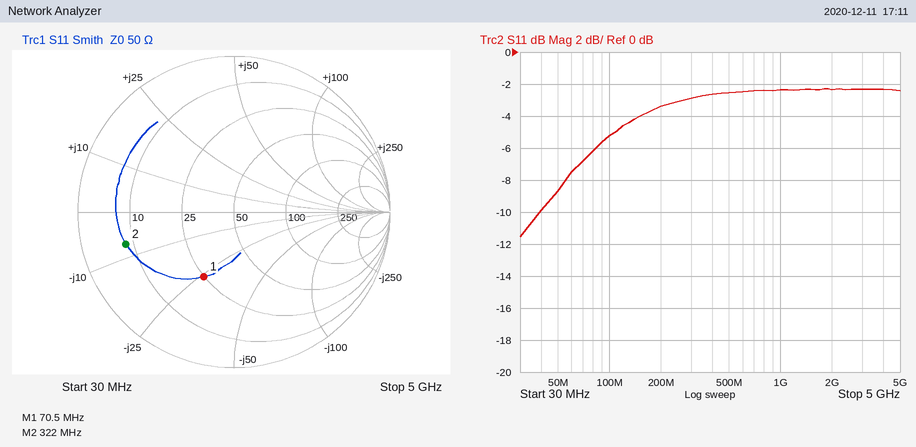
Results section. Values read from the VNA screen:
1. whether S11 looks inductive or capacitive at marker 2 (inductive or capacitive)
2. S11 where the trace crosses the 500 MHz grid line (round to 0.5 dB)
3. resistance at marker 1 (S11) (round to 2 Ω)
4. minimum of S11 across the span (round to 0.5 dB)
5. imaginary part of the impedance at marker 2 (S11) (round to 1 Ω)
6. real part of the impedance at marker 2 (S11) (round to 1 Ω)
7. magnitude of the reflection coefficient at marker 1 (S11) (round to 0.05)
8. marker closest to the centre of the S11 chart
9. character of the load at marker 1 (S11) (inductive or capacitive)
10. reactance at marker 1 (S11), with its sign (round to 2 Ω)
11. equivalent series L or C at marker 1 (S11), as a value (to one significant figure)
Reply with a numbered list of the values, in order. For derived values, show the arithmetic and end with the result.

1. capacitive
2. -2.5 dB
3. 24 Ω
4. -11.5 dB
5. -7 Ω
6. 8 Ω
7. 0.45
8. marker 1
9. capacitive
10. -26 Ω
11. C = 1/(2π × 70.5 MHz × 26 Ω) ≈ 86.8 pF, so 90 pF to one significant figure
